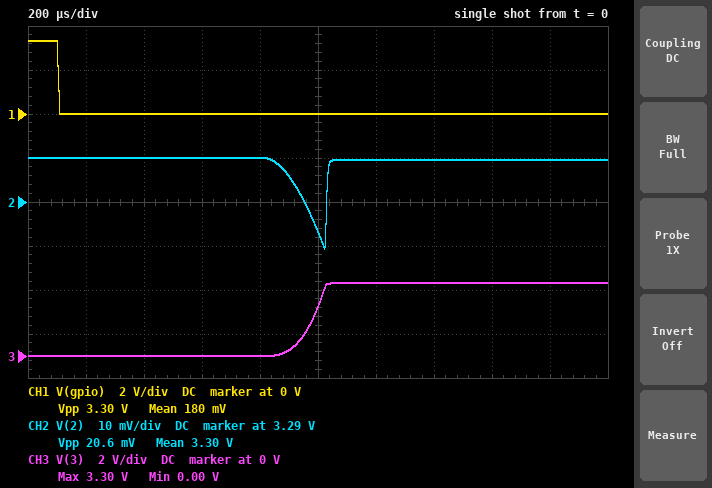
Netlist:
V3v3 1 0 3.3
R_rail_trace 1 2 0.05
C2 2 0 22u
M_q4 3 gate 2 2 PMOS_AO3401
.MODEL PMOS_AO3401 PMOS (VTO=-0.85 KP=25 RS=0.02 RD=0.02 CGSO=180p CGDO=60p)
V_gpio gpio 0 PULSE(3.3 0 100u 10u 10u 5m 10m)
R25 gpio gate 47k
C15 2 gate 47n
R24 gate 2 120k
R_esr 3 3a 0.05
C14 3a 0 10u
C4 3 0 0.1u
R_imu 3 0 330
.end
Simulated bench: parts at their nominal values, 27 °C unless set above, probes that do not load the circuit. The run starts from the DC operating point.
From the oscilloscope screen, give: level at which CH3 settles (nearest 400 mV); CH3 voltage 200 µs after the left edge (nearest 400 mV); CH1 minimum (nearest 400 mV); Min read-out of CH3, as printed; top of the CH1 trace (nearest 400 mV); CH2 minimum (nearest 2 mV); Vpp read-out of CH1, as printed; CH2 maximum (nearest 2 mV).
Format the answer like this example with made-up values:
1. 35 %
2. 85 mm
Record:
1. 3.2 V
2. 0 V
3. 0 V
4. 0.00 V
5. 3.2 V
6. 3.280 V
7. 3.30 V
8. 3.300 V
